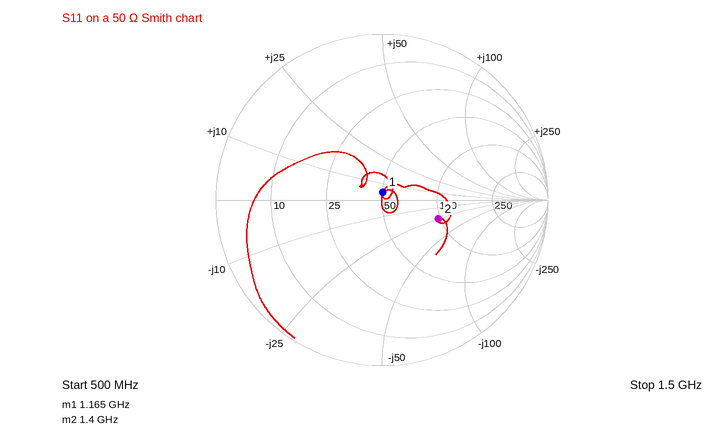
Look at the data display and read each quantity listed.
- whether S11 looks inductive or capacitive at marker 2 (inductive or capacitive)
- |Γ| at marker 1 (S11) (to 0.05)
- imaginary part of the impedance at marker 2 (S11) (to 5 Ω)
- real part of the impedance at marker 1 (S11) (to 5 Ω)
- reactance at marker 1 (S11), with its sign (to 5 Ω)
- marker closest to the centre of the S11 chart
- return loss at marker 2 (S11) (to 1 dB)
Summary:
capacitive
0.05
-25 Ω
50 Ω
+5 Ω
marker 1
9 dB
